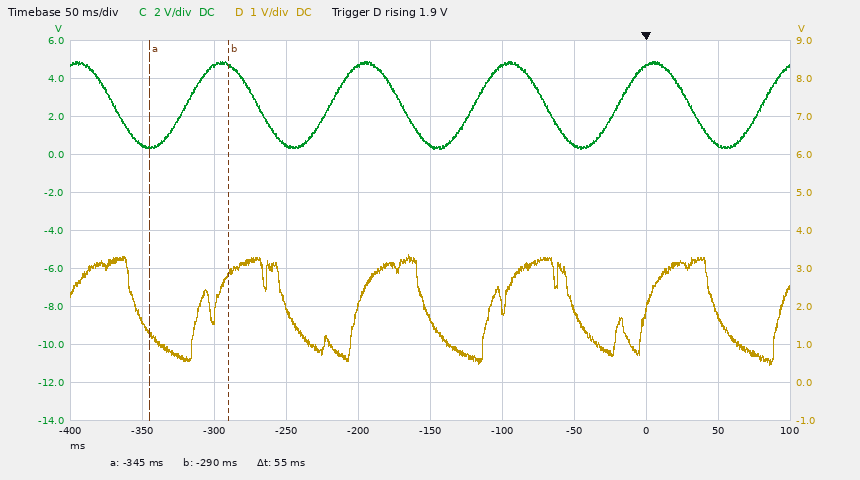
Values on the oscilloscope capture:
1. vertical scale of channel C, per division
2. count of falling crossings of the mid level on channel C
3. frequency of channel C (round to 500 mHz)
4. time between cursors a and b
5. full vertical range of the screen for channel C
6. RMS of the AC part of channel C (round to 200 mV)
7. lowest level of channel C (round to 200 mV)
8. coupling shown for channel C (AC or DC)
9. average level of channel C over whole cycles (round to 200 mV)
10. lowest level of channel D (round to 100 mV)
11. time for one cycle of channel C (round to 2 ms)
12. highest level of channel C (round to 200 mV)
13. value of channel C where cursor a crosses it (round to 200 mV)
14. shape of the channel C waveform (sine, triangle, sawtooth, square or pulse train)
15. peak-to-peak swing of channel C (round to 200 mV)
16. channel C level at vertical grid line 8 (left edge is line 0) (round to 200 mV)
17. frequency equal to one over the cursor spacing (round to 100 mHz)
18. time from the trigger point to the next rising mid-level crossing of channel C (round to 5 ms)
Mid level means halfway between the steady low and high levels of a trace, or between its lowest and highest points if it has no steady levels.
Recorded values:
2 V
5
10.0 Hz
55 ms
20 V
1.6 V
200 mV
DC
2.6 V
400 mV
100 ms
4.8 V
400 mV
sine
4.6 V
4.6 V
18.2 Hz
80 ms
